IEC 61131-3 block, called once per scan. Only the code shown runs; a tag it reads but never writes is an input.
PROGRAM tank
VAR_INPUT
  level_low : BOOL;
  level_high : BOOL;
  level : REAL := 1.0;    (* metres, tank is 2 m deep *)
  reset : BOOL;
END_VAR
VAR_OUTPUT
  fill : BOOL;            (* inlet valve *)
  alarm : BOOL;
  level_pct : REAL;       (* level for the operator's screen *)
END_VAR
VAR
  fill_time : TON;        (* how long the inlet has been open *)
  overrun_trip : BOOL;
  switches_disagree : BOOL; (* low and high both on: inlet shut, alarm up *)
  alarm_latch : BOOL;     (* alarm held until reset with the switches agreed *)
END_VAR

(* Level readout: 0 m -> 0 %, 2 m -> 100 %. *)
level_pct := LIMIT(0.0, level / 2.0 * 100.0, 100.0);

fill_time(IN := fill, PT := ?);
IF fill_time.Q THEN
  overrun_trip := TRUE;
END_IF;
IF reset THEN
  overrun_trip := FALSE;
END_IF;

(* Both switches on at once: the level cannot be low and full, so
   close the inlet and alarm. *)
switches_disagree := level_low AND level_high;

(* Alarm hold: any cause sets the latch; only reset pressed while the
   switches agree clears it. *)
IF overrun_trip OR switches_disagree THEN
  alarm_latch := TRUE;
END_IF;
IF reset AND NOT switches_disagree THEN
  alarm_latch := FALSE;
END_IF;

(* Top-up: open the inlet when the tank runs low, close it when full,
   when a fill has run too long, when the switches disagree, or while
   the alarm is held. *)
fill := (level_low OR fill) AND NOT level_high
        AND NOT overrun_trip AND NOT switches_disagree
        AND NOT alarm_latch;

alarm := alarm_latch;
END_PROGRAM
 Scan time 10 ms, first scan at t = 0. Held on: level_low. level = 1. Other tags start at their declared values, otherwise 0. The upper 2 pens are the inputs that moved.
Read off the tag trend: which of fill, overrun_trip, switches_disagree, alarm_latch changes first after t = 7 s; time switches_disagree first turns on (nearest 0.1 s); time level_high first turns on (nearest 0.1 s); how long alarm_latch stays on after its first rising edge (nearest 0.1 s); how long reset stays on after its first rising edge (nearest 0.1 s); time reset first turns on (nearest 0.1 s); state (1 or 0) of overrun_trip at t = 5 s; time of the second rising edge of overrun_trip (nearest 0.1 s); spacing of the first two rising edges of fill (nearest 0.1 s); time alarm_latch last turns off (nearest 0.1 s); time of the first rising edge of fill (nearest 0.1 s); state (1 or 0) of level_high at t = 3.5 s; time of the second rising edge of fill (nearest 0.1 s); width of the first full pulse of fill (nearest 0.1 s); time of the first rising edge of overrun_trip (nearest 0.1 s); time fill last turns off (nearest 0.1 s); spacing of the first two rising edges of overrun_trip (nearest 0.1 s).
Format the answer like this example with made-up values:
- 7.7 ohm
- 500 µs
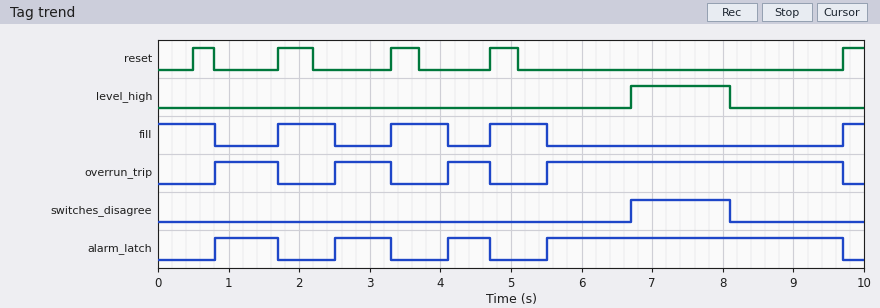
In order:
- switches_disagree
- 6.7 s
- 6.7 s
- 0.9 s
- 0.3 s
- 0.5 s
- 0
- 2.5 s
- 1.6 s
- 9.7 s
- 1.7 s
- 0
- 3.3 s
- 0.8 s
- 0.8 s
- 5.5 s
- 1.7 s
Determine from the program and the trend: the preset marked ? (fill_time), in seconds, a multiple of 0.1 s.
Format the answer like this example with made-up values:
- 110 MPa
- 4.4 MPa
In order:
- 0.8 s
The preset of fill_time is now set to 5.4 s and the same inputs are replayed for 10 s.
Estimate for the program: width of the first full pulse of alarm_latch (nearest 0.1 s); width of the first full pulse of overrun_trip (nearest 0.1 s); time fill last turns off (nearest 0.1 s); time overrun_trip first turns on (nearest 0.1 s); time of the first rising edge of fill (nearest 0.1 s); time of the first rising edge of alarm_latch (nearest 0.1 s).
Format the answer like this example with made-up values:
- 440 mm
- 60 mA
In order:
- 4.3 s
- 4.3 s
- 5.4 s
- 5.4 s
- 9.7 s
- 5.4 s
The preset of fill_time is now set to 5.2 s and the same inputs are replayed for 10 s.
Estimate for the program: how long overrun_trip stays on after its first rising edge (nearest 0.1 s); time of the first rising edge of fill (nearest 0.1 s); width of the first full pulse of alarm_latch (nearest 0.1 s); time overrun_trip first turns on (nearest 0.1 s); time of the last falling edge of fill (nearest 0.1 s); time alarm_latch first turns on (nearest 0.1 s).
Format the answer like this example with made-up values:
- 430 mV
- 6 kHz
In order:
- 4.5 s
- 9.7 s
- 4.5 s
- 5.2 s
- 5.2 s
- 5.2 s
